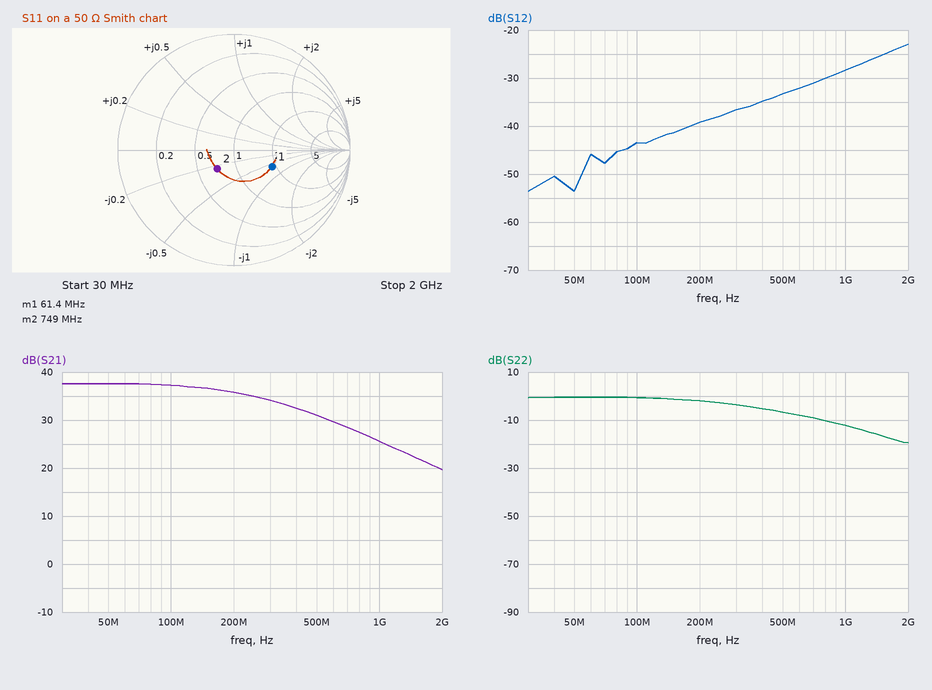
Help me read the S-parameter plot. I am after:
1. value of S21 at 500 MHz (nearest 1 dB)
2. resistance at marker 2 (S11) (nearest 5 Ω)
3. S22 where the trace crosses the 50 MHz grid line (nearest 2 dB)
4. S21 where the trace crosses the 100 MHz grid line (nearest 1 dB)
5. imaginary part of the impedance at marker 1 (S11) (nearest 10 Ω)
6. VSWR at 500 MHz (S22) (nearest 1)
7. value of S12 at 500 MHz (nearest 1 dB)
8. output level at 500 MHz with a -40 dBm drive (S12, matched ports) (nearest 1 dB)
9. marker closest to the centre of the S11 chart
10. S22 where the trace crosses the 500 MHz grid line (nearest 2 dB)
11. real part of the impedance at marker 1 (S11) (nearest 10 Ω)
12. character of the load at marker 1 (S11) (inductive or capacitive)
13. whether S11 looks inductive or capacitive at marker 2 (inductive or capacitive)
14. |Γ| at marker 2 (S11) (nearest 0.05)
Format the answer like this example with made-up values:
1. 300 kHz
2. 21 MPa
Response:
1. 31 dB
2. 35 Ω
3. 0 dB
4. 37 dB
5. -30 Ω
6. 3
7. -33 dB
8. -73 dBm
9. marker 2
10. -6 dB
11. 90 Ω
12. capacitive
13. capacitive
14. 0.20
